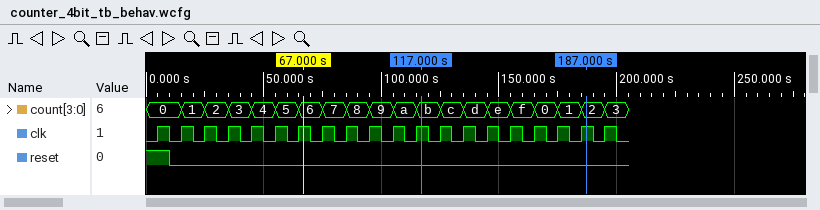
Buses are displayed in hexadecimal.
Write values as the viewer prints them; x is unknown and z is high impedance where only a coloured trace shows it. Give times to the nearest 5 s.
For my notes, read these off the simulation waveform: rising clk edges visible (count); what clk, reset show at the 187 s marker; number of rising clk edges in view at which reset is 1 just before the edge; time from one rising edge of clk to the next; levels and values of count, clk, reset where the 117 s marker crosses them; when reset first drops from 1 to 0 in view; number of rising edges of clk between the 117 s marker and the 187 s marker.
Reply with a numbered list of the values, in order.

1. 20
2. clk=1, reset=0
3. 1
4. 10 s
5. count=b, clk=1, reset=0
6. 10 s
7. 7
